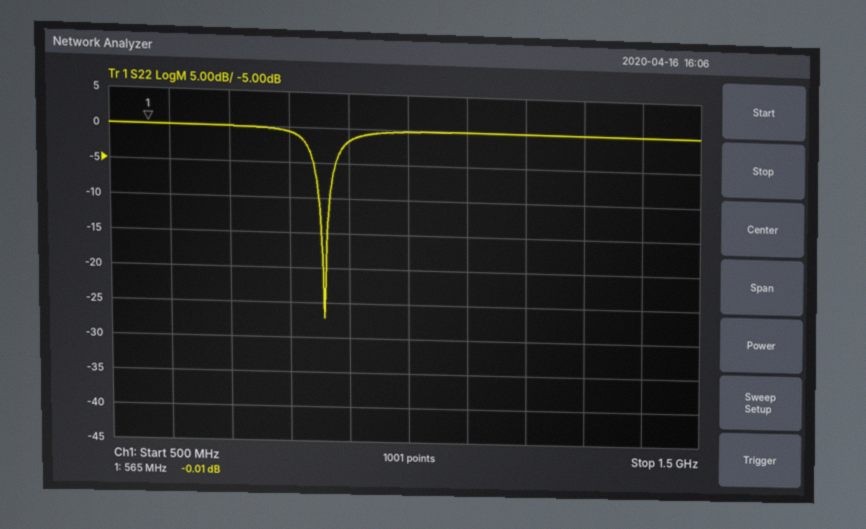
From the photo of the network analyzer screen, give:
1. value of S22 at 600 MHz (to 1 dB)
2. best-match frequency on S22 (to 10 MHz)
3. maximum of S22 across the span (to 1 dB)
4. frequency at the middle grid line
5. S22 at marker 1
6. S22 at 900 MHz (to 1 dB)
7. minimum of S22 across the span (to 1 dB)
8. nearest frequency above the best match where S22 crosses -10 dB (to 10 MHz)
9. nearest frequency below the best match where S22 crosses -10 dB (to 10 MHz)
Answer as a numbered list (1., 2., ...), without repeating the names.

1. 0 dB
2. 860 MHz
3. 0 dB
4. 1 GHz
5. -0.01 dB
6. -2 dB
7. -27 dB
8. 870 MHz
9. 850 MHz
